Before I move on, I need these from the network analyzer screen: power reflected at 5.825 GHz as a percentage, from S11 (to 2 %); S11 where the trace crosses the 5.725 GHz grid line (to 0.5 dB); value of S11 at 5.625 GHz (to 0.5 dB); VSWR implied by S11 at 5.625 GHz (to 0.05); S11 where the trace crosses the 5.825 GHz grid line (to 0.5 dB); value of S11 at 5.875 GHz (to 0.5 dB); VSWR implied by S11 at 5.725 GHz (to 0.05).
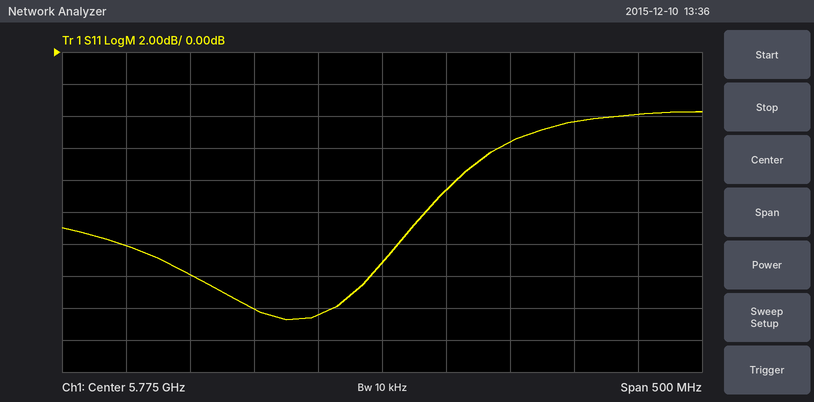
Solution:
14 %
-16.5 dB
-14.0 dB
1.50
-8.5 dB
-5.5 dB
1.35
